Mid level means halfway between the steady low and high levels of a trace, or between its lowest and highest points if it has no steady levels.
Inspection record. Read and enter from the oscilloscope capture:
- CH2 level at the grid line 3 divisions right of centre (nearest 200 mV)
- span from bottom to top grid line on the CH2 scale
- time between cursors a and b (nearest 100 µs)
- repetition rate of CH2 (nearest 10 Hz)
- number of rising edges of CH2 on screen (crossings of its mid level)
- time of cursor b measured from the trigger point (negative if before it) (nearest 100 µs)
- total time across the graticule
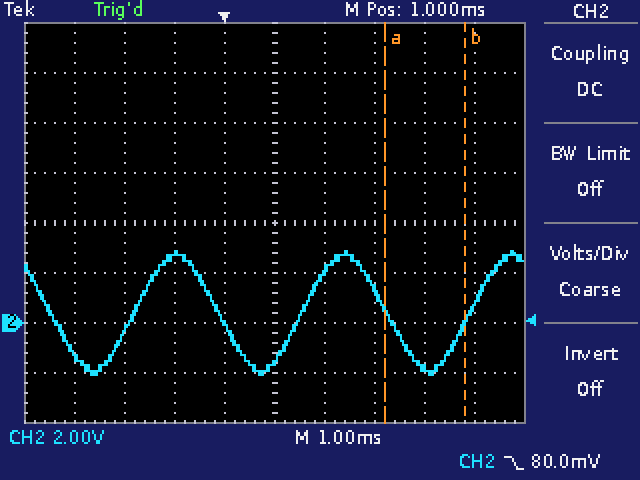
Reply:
-1.8 V
16 V
1.6 ms
300 Hz
3
+4.8 ms
10 ms
